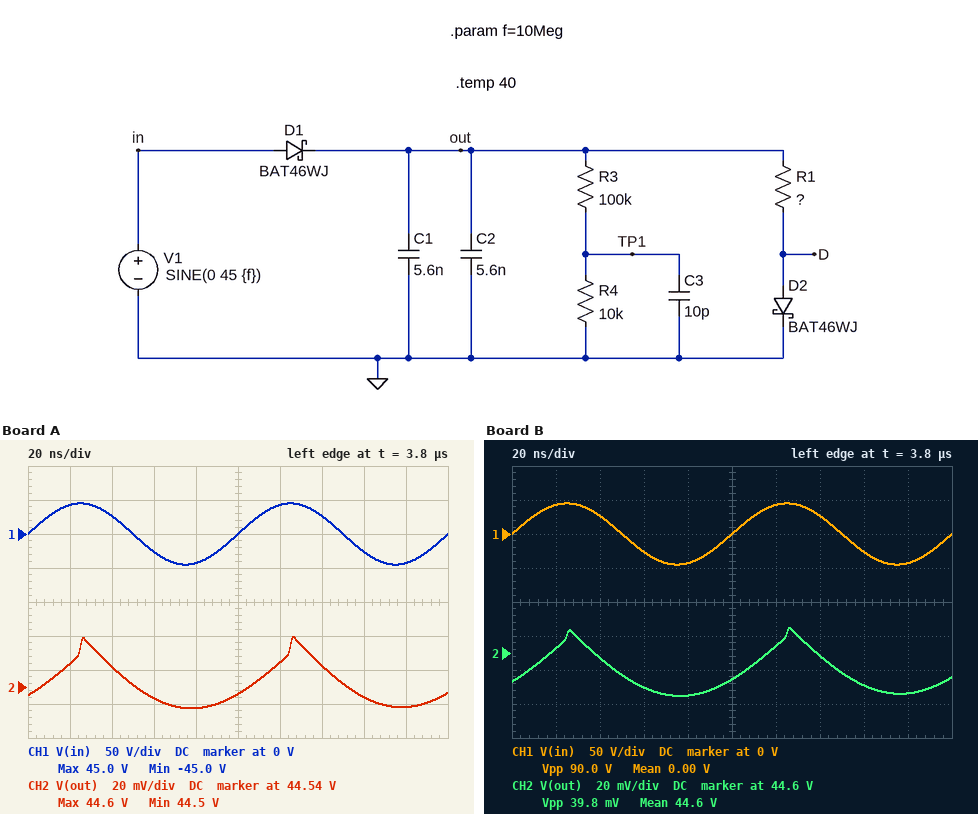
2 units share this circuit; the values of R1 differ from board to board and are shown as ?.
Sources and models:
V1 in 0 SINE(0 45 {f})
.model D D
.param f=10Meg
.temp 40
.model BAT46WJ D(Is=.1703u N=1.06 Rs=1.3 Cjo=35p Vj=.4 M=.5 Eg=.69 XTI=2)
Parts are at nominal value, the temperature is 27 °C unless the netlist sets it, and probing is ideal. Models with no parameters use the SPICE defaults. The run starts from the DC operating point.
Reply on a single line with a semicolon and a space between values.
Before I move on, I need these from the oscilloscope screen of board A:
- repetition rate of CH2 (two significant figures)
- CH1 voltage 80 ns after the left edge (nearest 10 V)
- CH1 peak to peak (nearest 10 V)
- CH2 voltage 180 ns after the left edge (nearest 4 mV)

10 MHz; -40 V; 90 V; 44.528 V
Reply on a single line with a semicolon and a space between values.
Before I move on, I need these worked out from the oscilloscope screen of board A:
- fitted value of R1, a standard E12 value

56 kΩ
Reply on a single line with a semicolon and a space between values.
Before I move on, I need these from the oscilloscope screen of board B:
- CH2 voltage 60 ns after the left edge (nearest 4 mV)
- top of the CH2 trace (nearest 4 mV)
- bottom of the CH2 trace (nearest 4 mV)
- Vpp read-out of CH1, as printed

44.580 V; 44.616 V; 44.576 V; 90.0 V
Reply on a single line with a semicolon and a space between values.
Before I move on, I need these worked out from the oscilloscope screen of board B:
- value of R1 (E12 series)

270 kΩ
